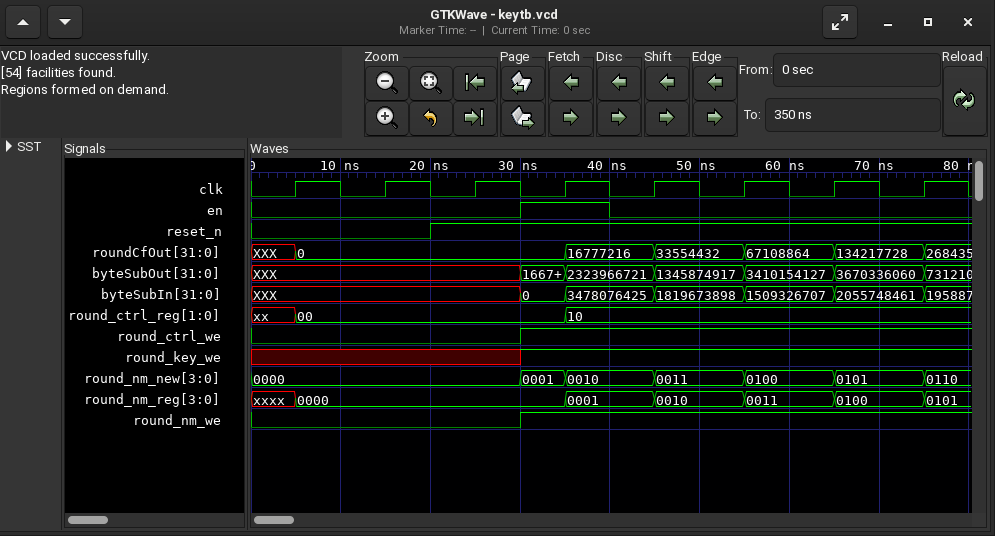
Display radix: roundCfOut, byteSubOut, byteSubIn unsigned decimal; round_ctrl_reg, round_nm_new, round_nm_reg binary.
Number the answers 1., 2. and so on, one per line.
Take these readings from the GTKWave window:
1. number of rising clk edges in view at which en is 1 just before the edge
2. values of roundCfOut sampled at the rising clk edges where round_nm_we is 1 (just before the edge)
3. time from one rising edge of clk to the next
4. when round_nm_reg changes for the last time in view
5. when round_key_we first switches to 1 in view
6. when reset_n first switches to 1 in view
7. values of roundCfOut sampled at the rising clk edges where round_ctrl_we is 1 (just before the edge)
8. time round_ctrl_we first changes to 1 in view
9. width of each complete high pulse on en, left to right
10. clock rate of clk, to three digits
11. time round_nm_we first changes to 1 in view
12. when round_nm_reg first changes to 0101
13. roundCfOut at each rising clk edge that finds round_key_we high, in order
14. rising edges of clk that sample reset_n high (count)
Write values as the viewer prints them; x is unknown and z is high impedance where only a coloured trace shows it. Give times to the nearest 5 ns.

1. 1
2. 0, 16777216, 33554432, 67108864, 134217728
3. 10 ns
4. 75 ns
5. 30 ns
6. 20 ns
7. 0, 16777216, 33554432, 67108864, 134217728
8. 30 ns
9. 10 ns
10. 100 MHz
11. 30 ns
12. 75 ns
13. 0, 16777216, 33554432, 67108864, 134217728
14. 6
